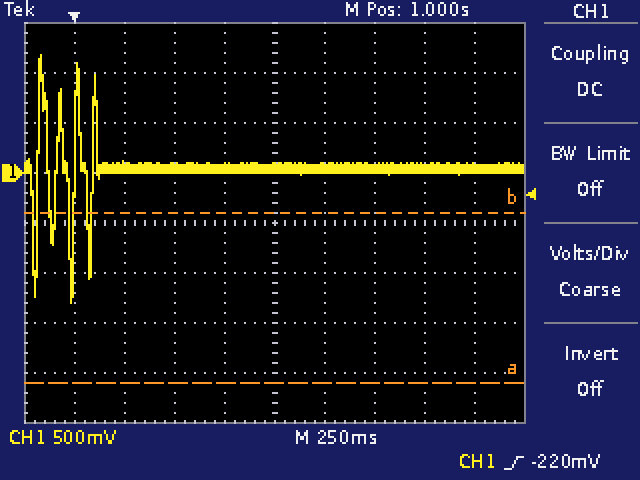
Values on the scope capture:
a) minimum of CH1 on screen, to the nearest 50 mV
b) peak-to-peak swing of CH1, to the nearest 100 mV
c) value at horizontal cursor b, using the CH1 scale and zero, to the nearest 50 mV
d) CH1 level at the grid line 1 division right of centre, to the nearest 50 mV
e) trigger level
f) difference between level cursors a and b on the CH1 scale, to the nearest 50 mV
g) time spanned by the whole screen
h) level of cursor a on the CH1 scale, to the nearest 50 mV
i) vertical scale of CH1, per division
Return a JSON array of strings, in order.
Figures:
["-1.30 V", "2.50 V", "-400 mV", "50 mV", "-220 mV", "1.70 V", "2.5 s", "-2.10 V", "500 mV"]
